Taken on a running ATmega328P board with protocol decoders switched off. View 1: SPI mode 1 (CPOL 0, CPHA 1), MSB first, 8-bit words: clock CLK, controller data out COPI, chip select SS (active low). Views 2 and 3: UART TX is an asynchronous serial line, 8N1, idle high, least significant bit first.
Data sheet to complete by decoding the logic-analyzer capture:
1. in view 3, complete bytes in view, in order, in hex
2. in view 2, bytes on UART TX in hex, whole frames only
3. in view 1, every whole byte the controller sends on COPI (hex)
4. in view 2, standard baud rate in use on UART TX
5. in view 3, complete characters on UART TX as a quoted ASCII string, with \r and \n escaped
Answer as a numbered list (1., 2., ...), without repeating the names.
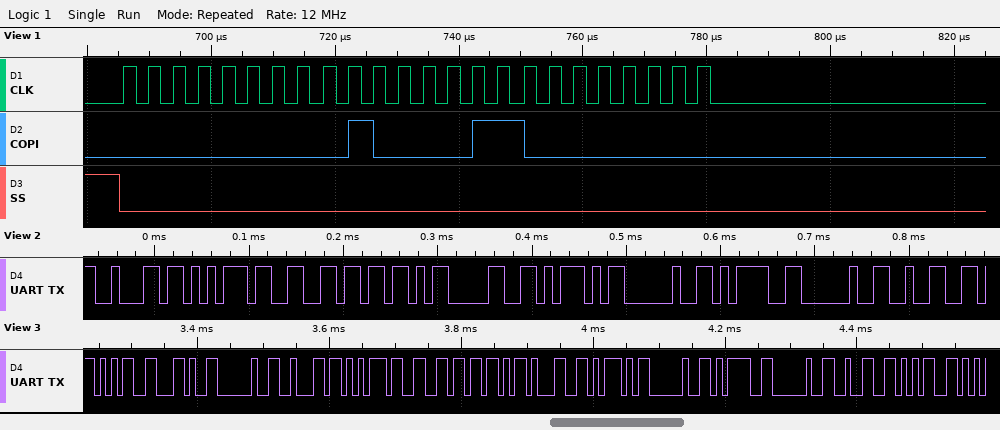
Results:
1. 35 2C 20 62 75 66 5B 31 5D 20 3D 20 32 35
2. 62 75 66 5B 30 5D 20 3D 20 32
3. 00 43 00
4. 115200 baud
5. "5, buf[1] = 25"
